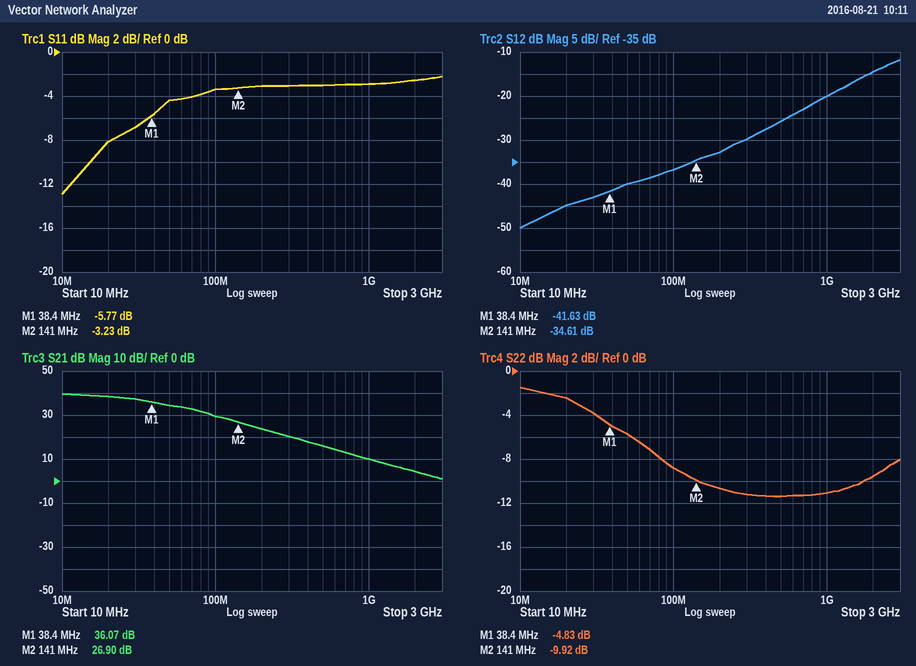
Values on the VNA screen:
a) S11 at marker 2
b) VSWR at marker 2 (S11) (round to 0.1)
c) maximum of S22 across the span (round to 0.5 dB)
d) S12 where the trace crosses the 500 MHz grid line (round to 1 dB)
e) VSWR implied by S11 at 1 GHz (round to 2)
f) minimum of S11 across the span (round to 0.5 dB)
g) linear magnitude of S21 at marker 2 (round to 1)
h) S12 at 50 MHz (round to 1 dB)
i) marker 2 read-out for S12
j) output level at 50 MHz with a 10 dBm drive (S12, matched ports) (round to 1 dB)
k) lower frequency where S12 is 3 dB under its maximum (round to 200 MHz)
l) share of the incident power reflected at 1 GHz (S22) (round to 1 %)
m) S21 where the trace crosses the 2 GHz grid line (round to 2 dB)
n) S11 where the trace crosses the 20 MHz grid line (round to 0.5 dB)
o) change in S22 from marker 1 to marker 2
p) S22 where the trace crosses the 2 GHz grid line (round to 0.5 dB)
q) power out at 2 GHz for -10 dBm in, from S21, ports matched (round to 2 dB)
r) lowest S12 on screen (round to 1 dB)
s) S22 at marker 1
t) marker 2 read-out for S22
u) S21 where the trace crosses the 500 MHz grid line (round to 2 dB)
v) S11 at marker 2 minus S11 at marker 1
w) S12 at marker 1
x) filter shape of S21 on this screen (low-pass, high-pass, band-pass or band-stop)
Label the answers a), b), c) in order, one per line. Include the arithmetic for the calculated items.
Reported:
a) -3.23 dB
b) (1 + 0.6894)/(1 − 0.6894) ≈ 5.4
c) -1.5 dB
d) -26 dB
e) |Γ| = 10^(-3/20) = 0.7079; VSWR = (1 + 0.7079)/(1 − 0.7079) ≈ 6
f) -13.0 dB
g) 10^(26.9/20) ≈ 22
h) -40 dB
i) -34.61 dB
j) 10 dBm + (-40 dB) = -30 dBm
k) 2.0 GHz
l) 10^(-11/10) ≈ 8 %
m) 4 dB
n) -8.0 dB
o) -9.92 − (-4.83) = -5.09 dB
p) -9.5 dB
q) -10 dBm + (4 dB) = -6 dBm
r) -50 dB
s) -4.83 dB
t) -9.92 dB
u) 16 dB
v) -3.23 − (-5.77) = 2.54 dB
w) -41.63 dB
x) low-pass
